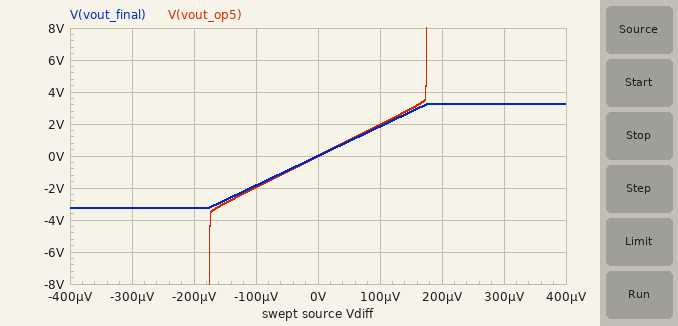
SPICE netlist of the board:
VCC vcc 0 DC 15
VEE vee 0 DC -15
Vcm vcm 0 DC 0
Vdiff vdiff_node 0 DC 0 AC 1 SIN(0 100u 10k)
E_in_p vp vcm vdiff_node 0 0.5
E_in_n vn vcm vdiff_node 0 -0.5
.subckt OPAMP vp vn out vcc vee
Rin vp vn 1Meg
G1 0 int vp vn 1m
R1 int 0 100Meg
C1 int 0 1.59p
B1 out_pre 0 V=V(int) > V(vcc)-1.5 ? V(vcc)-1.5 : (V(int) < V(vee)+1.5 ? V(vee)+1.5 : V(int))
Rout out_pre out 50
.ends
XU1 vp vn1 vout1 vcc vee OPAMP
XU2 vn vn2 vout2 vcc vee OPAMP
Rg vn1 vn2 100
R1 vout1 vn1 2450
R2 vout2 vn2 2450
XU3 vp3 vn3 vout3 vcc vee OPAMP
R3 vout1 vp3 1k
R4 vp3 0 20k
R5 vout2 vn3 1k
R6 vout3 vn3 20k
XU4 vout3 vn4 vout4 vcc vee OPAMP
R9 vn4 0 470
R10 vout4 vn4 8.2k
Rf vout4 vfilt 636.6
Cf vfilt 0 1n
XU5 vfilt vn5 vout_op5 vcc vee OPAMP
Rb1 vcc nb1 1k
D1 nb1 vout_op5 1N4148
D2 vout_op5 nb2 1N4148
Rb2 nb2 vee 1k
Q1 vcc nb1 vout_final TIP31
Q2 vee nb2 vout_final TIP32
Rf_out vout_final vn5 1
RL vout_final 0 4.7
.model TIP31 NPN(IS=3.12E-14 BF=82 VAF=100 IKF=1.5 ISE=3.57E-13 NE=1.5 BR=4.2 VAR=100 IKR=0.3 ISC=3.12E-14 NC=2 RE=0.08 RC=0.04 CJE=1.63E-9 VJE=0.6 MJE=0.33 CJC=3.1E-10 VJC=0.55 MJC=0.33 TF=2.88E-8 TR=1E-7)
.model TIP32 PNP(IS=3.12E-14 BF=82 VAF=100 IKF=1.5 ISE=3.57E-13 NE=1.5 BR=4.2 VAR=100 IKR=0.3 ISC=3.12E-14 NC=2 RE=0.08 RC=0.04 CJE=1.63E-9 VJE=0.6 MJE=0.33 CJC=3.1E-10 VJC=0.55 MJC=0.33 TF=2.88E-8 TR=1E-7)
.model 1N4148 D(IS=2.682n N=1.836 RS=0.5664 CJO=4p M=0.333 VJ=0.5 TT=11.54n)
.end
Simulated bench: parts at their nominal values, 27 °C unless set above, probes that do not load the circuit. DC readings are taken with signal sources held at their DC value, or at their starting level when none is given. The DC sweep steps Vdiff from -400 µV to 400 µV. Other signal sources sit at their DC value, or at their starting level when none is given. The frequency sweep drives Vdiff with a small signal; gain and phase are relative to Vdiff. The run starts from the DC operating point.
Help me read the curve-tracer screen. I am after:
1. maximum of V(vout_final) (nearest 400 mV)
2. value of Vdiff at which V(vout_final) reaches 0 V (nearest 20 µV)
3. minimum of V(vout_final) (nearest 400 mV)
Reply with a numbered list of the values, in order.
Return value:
1. 3.2 V
2. 0 V
3. -3.2 V
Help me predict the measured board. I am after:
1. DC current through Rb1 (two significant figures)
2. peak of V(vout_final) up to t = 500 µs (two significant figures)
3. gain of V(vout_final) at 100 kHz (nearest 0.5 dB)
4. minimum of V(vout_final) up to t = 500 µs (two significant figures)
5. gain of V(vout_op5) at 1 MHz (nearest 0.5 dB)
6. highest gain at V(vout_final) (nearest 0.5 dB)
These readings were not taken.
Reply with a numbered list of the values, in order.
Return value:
1. 14 mA
2. 1.8 V
3. 84.5 dB
4. -1.8 V
5. 72.5 dB
6. 85.5 dB
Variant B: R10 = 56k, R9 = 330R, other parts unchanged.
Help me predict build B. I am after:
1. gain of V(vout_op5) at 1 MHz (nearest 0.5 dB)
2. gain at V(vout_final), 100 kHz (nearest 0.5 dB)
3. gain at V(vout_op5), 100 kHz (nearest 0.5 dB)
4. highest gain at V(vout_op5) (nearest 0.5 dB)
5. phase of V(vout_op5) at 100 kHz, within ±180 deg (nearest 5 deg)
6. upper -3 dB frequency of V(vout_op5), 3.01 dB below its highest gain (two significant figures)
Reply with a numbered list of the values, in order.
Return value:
1. 85.5 dB
2. 104.0 dB
3. 104.5 dB
4. 105.0 dB
5. -35 deg
6. 220 kHz
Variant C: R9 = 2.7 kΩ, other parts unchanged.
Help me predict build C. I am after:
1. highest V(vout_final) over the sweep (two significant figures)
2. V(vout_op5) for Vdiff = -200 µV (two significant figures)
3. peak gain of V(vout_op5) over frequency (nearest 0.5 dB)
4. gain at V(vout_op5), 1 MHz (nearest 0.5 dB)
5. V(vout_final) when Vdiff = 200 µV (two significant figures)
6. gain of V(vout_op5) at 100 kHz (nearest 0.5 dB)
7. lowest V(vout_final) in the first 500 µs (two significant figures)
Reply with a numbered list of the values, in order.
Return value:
1. 1.6 V
2. -850 mV
3. 72.5 dB
4. 59.5 dB
5. 810 mV
6. 72.0 dB
7. -400 mV
